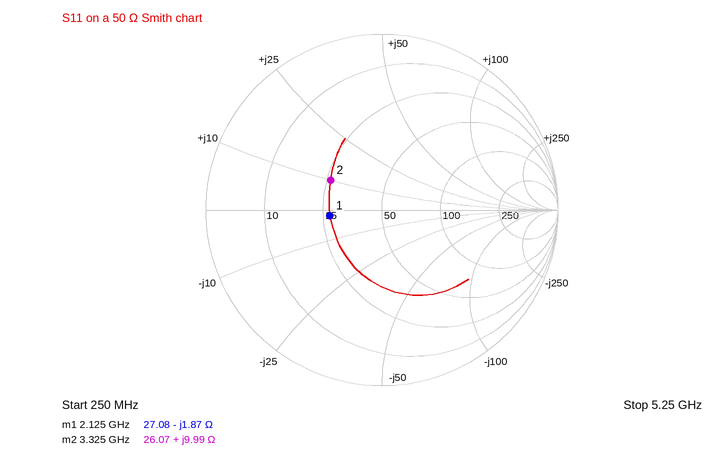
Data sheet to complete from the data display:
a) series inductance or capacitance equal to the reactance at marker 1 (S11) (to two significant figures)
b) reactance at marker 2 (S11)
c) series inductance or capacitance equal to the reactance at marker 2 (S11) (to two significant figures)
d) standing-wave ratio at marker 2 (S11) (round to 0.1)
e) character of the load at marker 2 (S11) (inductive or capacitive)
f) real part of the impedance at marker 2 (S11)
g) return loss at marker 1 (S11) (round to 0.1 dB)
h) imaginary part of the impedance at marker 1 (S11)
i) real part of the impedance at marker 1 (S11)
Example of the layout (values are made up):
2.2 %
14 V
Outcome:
40 pF
+9.99 Ω
480 pH
2.0
inductive
26.07 Ω
10.5 dB
-1.87 Ω
27.08 Ω
